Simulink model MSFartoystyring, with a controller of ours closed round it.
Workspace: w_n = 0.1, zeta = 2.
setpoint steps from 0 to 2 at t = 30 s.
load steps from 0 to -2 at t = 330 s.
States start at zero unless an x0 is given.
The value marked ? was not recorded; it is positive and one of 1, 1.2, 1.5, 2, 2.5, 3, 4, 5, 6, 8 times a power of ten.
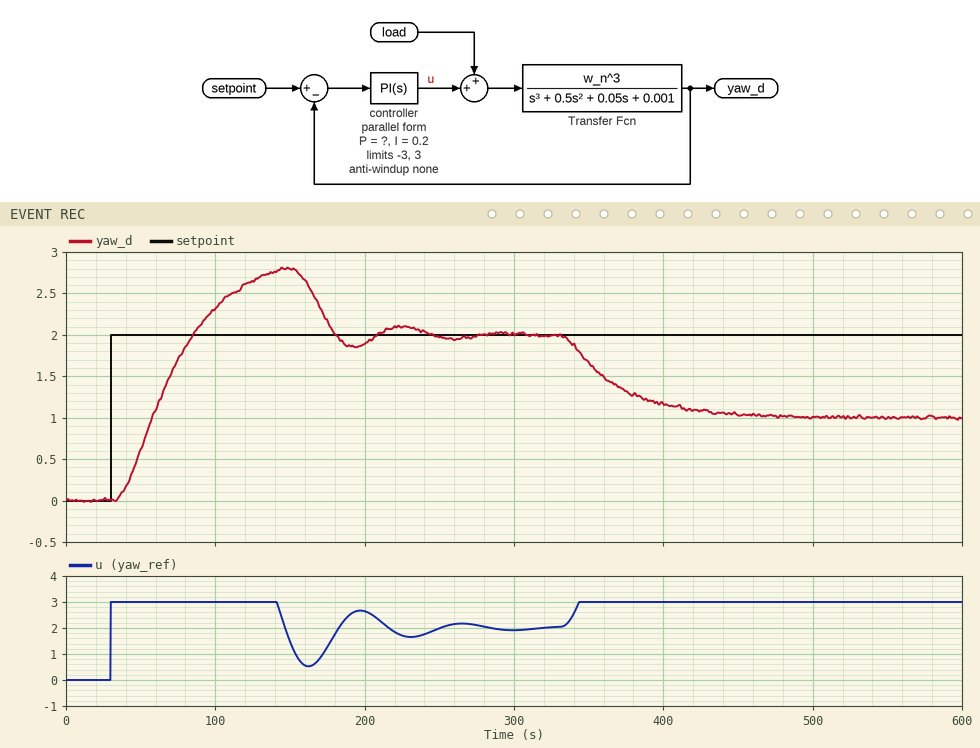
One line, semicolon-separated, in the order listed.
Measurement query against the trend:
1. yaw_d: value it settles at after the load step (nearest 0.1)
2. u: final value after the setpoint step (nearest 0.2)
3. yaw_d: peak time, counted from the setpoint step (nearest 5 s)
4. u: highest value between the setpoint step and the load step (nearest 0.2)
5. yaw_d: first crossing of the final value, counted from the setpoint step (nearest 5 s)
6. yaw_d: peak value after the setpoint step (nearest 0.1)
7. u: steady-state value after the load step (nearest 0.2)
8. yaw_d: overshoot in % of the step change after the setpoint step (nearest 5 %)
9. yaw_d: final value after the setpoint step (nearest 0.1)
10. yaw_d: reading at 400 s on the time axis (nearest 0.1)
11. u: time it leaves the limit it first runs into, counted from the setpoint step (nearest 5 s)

1.0; 2.0; 120 s; 3.0; 55 s; 2.8; 3.0; 40 %; 2.0; 1.2; 110 s
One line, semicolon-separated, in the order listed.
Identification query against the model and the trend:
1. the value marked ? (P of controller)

4
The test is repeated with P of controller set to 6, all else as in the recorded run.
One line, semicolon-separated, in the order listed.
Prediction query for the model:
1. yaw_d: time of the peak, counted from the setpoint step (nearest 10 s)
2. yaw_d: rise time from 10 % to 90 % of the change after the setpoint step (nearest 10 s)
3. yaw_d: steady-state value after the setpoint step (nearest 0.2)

110 s; 40 s; 2.0
